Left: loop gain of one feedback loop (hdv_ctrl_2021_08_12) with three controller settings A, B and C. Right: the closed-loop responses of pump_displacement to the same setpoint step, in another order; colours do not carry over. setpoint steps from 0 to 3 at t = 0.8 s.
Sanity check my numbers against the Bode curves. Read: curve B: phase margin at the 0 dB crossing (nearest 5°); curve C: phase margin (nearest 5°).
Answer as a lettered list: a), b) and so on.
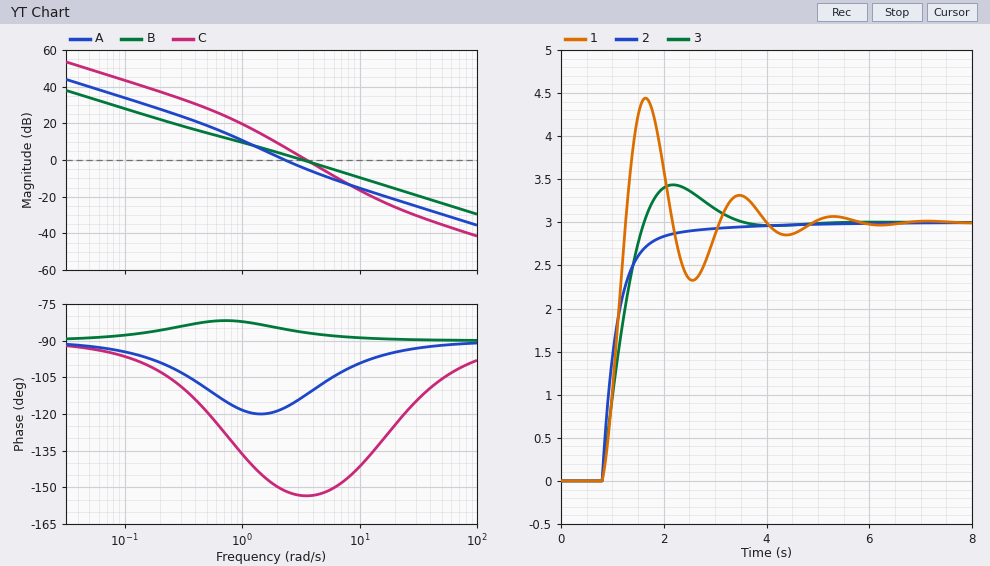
a) 95°
b) 25°
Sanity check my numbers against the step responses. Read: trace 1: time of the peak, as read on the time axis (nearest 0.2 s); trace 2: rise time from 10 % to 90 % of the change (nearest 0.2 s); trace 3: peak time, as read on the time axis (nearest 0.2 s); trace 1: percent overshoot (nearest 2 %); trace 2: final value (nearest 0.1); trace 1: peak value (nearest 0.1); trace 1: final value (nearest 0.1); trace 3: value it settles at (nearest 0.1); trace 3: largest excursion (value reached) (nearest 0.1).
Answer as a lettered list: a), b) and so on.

a) 1.6 s
b) 0.8 s
c) 2.2 s
d) 48 %
e) 3.0
f) 4.4
g) 3.0
h) 3.0
i) 3.4
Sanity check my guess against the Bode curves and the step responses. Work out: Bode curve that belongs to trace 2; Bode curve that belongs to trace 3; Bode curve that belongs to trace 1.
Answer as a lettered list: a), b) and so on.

a) B
b) A
c) C
